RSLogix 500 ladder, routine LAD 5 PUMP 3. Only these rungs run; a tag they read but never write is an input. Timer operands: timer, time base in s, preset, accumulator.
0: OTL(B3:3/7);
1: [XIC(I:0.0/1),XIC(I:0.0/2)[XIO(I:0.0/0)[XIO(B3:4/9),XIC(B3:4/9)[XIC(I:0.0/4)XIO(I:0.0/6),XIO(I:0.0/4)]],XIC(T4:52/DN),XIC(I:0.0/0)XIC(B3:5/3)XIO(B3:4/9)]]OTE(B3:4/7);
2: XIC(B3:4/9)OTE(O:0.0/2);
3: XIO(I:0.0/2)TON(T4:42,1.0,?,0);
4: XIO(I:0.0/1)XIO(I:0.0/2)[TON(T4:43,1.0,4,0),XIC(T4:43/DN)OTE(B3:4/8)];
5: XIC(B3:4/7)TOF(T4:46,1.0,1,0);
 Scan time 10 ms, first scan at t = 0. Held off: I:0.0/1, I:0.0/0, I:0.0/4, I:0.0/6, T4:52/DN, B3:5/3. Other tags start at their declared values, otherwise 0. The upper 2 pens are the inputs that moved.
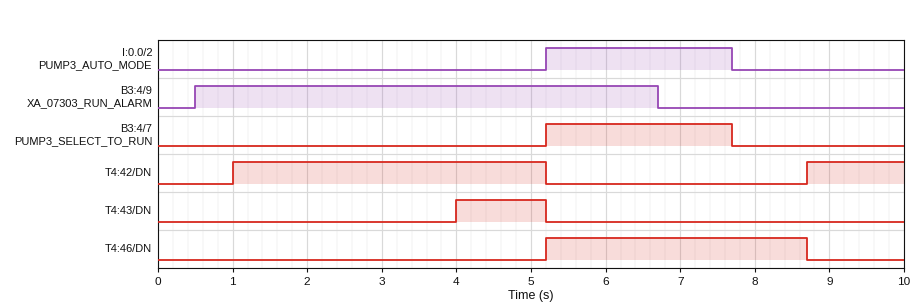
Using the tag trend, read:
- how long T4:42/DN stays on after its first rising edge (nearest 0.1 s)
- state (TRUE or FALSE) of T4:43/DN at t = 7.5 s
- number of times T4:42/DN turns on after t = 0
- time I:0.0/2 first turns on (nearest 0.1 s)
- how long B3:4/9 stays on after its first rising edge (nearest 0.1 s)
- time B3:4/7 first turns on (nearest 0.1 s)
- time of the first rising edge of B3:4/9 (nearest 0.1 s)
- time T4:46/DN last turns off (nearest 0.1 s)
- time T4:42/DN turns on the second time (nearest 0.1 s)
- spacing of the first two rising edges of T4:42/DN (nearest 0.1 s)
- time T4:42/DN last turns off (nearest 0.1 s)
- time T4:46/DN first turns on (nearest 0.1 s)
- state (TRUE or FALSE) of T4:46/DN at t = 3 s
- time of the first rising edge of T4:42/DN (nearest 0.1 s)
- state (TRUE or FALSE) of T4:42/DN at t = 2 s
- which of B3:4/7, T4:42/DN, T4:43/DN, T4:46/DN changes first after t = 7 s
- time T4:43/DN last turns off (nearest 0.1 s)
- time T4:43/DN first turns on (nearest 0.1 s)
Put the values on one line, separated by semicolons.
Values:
4.2 s; FALSE; 2; 5.2 s; 6.2 s; 5.2 s; 0.5 s; 8.7 s; 8.7 s; 7.7 s; 5.2 s; 5.2 s; FALSE; 1.0 s; TRUE; B3:4/7; 5.2 s; 4.0 s
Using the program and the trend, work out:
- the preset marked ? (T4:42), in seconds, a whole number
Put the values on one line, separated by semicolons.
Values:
1 s
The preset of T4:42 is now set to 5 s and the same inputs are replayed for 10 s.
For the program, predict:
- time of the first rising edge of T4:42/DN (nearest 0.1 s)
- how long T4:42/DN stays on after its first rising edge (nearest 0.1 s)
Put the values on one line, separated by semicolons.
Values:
5.0 s; 0.2 s
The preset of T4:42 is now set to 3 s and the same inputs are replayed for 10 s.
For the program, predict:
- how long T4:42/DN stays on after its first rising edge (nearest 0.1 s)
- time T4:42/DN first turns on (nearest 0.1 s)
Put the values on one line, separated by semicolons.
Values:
2.2 s; 3.0 s
